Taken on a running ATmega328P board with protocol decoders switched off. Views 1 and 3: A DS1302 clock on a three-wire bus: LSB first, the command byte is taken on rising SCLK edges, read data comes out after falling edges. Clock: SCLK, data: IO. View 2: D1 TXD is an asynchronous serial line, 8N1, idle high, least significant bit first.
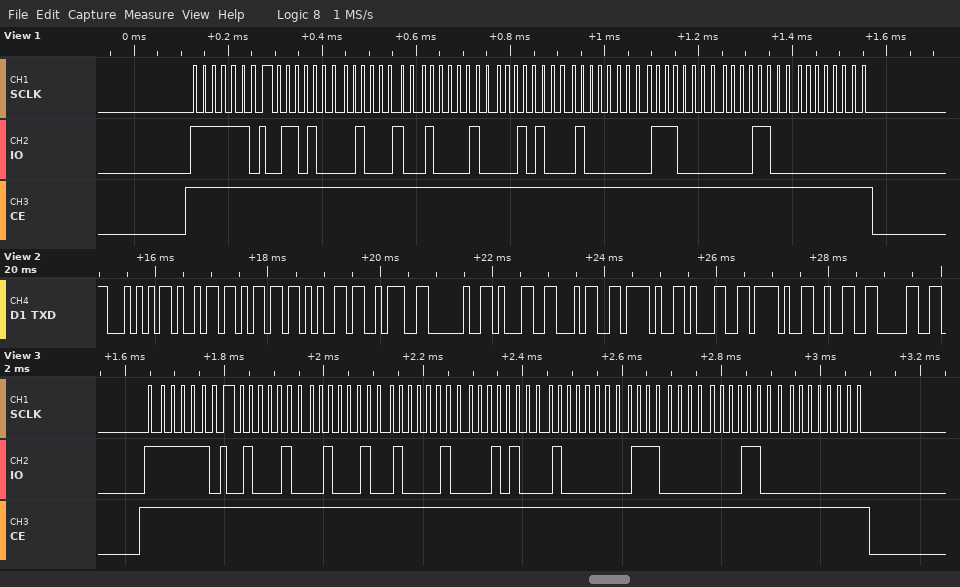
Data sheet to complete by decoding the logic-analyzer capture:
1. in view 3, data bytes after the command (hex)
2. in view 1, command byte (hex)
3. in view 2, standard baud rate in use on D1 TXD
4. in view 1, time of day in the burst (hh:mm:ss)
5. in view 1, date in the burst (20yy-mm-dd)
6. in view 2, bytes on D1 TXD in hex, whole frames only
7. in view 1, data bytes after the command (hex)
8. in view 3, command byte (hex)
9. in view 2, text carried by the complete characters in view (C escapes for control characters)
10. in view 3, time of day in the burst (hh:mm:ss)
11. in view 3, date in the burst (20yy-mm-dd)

22 22 21 14 01 07 18 00
0xBF
9600 baud
21:22:16
2018-01-14
0x54 0x69 0x6D 0x65 0x3A 0x20 0x31 0x34 0x2F 0x31 0x2F 0x32 0x30
16 22 21 14 01 07 18 00
0xBF
"Time: 14/1/20"
21:22:22
2018-01-14
